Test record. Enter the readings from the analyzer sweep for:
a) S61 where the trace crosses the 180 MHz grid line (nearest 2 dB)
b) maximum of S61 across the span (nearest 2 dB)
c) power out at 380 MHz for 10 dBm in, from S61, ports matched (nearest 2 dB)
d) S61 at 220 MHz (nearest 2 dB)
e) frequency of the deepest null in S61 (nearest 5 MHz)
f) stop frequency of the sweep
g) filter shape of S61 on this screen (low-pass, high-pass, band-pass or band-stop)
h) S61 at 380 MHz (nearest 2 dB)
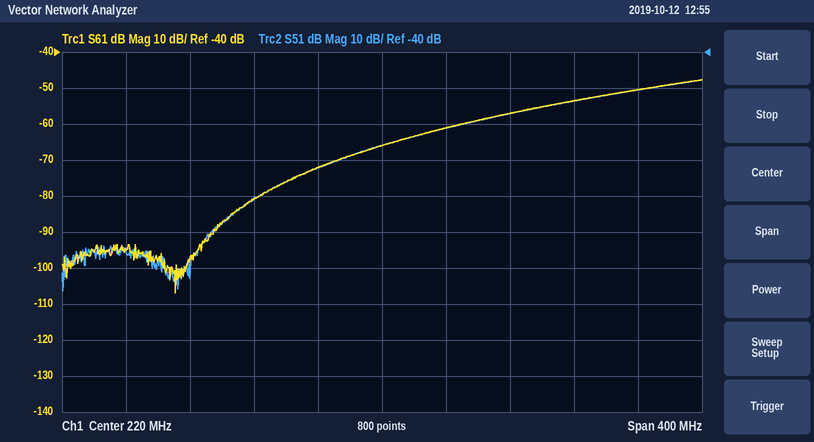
-72 dB
-48 dB
-40 dBm
-66 dB
90 MHz
420 MHz
high-pass
-50 dB
